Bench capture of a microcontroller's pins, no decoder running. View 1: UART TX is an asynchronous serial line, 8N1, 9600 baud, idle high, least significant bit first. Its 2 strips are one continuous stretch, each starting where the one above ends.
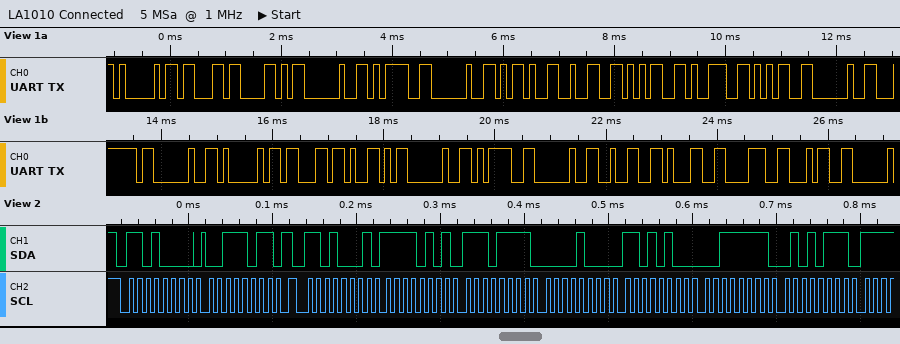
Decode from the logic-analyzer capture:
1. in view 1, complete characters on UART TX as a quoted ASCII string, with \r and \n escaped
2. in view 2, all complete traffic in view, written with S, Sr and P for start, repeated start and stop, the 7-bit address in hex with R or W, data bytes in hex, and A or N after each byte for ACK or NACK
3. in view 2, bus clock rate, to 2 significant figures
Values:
"AcX = -2595 | AcY = 2184"
S 68W A 3B A Sr 68R A F5 A EF A 08 A D4 A 3F A 57 A
100 kHz
